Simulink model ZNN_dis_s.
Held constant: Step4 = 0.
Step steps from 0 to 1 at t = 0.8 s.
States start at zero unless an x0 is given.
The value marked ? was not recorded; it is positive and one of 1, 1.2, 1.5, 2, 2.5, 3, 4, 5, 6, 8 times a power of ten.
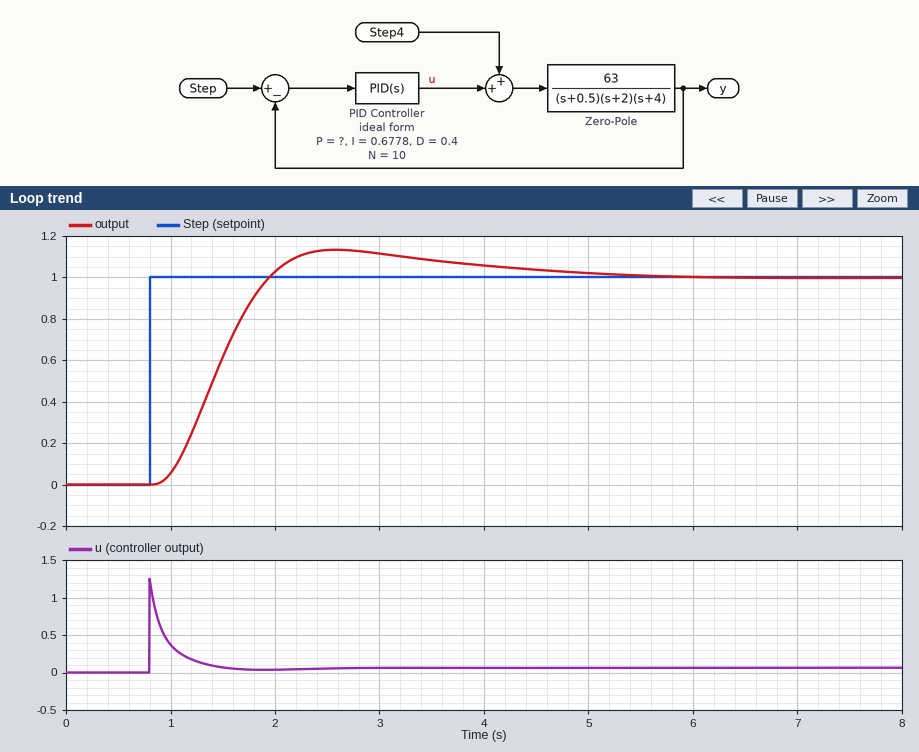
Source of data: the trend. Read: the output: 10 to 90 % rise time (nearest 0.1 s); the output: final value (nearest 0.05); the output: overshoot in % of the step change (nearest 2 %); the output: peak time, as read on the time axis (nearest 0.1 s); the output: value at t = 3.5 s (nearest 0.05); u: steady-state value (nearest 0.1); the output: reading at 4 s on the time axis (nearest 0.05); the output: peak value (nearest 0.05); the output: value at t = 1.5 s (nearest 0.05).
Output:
0.7 s
1.00
14 %
2.6 s
1.10
0.1
1.05
1.15
0.60
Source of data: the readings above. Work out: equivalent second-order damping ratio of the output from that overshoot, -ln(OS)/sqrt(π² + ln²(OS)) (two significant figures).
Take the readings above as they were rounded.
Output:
0.53
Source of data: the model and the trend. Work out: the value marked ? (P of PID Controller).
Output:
0.25
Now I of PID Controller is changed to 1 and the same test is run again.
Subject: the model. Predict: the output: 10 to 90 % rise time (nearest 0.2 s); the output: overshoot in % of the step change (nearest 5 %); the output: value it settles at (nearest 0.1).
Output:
0.6 s
25 %
1.0
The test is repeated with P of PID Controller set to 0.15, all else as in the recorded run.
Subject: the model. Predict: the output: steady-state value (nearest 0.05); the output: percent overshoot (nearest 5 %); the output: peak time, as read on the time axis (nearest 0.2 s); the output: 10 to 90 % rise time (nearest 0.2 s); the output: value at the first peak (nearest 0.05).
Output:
1.00
10 %
4.0 s
1.2 s
1.10
